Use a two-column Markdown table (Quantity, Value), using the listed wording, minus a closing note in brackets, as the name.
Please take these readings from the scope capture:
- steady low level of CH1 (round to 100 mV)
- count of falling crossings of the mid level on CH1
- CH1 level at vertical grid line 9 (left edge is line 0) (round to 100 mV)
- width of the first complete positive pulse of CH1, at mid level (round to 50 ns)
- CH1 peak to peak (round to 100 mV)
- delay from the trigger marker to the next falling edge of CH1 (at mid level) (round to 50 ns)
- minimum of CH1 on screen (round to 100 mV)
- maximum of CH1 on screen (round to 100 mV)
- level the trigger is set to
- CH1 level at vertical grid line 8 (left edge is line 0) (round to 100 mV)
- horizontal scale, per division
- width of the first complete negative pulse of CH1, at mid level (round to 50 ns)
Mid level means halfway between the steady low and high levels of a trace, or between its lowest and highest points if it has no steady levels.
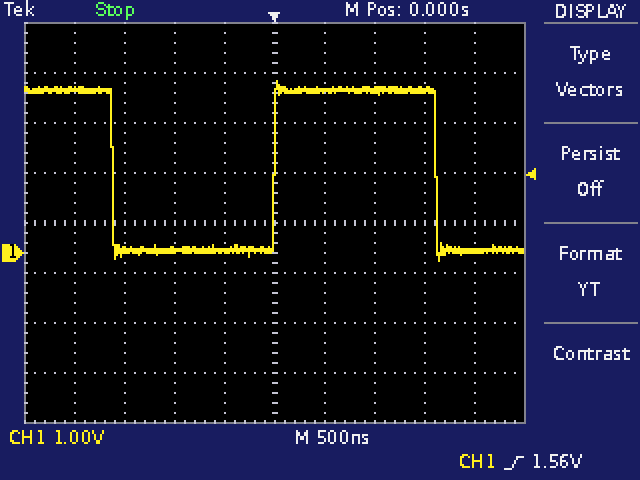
| Quantity | Value |
|---|---|
| steady low level of CH1 | 0.0 V |
| count of falling crossings of the mid level on CH1 | 2 |
| CH1 level at vertical grid line 9 (left edge is line 0) | 0.0 V |
| width of the first complete positive pulse of CH1, at mid level | 1.60 µs |
| CH1 peak to peak | 3.6 V |
| delay from the trigger marker to the next falling edge of CH1 (at mid level) | 1.60 µs |
| minimum of CH1 on screen | -200 mV |
| maximum of CH1 on screen | 3.4 V |
| level the trigger is set to | 1.56 V |
| CH1 level at vertical grid line 8 (left edge is line 0) | 3.3 V |
| horizontal scale, per division | 500 ns |
| width of the first complete negative pulse of CH1, at mid level | 1.60 µs |
